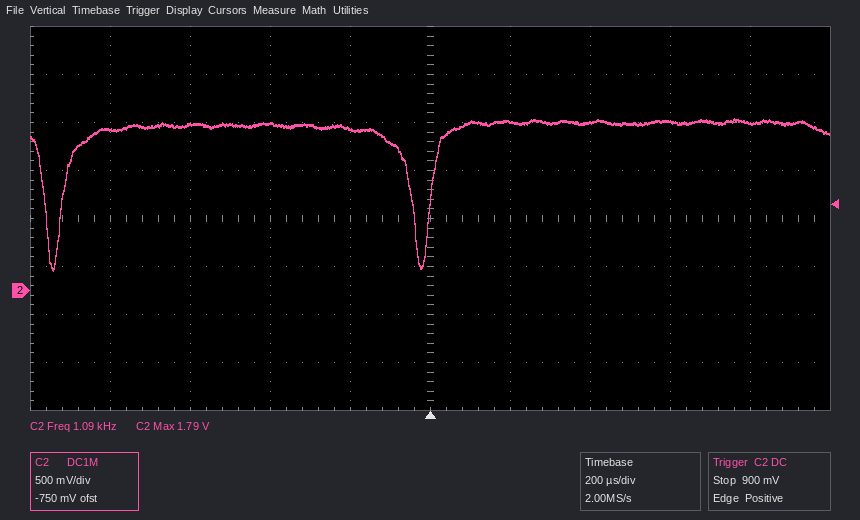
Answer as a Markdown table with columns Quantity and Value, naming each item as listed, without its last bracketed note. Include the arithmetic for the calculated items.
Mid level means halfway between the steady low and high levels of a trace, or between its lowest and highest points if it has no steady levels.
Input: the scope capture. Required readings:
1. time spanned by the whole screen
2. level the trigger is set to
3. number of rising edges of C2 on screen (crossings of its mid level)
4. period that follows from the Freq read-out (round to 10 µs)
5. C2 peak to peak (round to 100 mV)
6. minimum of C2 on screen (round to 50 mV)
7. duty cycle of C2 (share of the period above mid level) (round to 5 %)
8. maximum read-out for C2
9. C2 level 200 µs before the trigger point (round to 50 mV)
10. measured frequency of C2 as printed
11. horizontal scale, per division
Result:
| Quantity | Value |
|---|---|
| time spanned by the whole screen | 2 ms |
| level the trigger is set to | 900 mV |
| number of rising edges of C2 on screen | 2 |
| period that follows from the Freq read-out | 1 / 1.09 kHz ≈ 917 µs, so 920 µs to the nearest 10 µs |
| C2 peak to peak | 1.60 V |
| minimum of C2 on screen | 200 mV |
| duty cycle of C2 (share of the period above mid level) | 95 % |
| maximum read-out for C2 | 1.79 V |
| C2 level 200 µs before the trigger point | 1.70 V |
| measured frequency of C2 as printed | 1.09 kHz |
| horizontal scale, per division | 200 µs |
